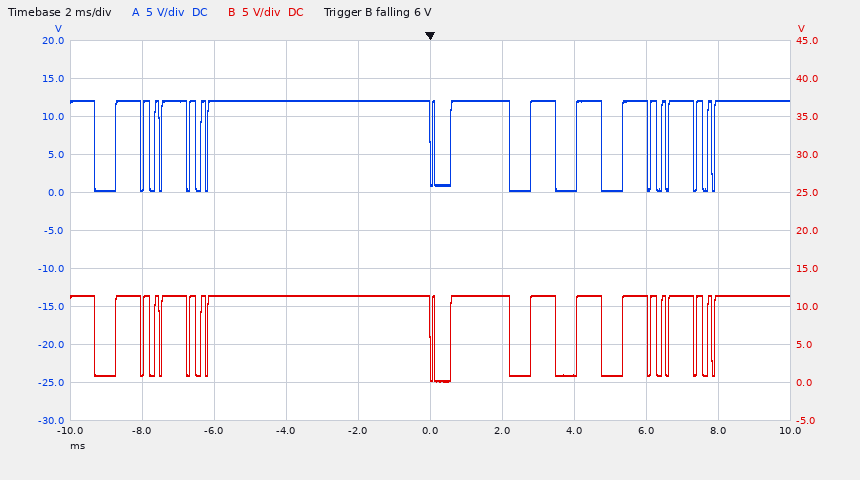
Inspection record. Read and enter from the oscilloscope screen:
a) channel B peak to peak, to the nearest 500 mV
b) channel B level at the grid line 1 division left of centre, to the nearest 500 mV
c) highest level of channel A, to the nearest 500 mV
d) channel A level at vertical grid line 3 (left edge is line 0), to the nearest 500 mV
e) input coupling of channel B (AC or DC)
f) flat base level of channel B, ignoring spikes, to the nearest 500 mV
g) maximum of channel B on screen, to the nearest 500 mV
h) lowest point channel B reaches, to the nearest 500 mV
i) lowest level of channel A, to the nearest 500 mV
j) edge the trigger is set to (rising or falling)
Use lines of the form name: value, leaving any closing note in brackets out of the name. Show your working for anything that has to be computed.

channel B peak to peak, to the nearest 500 mV: 11.5 V − (0.0 V) = 11.5 V
channel B level at the grid line 1 division left of centre, to the nearest 500 mV: 11.5 V
highest level of channel A, to the nearest 500 mV: 12.0 V
channel A level at vertical grid line 3 (left edge is line 0), to the nearest 500 mV: 12.0 V
input coupling of channel B: DC
flat base level of channel B, ignoring spikes, to the nearest 500 mV: 1.0 V
maximum of channel B on screen, to the nearest 500 mV: 11.5 V
lowest point channel B reaches, to the nearest 500 mV: 0.0 V
lowest level of channel A, to the nearest 500 mV: 500 mV
edge the trigger is set to: falling
